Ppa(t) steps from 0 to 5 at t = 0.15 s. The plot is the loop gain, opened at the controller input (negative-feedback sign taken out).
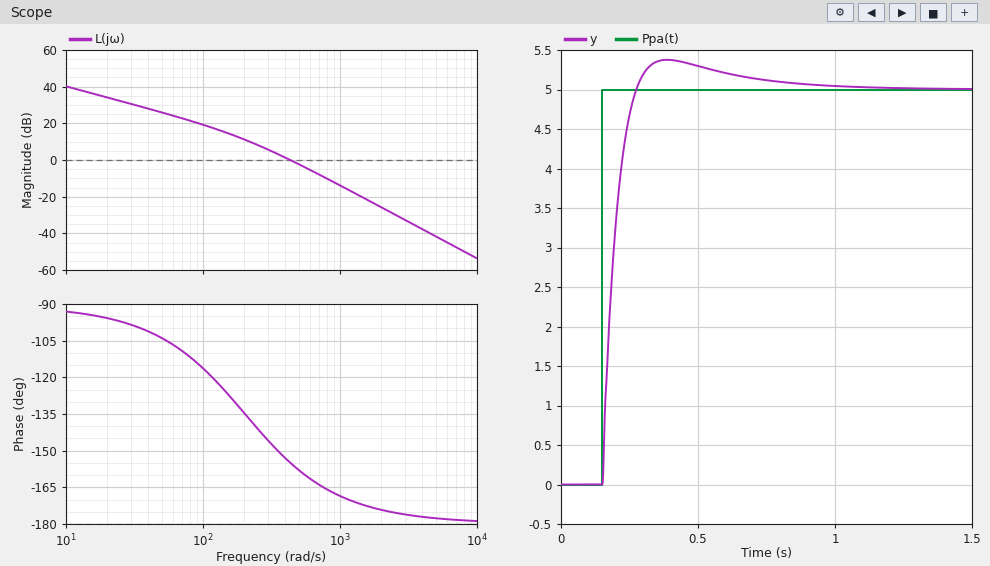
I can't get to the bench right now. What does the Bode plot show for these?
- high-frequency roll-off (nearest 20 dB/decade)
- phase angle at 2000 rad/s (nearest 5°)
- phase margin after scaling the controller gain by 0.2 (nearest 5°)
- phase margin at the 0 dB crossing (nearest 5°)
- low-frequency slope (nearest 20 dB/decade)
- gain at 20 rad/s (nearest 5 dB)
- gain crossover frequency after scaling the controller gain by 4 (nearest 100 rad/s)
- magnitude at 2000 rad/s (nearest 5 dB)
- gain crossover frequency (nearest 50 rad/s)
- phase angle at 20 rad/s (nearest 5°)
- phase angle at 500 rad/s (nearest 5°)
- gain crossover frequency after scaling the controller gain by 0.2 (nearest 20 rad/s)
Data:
-40 dB/decade
-175°
50°
25°
-20 dB/decade
35 dB
900 rad/s
-25 dB
450 rad/s
-95°
-160°
160 rad/s
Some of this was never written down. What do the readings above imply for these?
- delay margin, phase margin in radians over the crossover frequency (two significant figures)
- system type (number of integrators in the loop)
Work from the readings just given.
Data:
0.00097 s
1
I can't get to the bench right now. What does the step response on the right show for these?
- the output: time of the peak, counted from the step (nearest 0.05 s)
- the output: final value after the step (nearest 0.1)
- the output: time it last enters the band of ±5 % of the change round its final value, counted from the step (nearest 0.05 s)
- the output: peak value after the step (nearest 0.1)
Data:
0.25 s
5.0
0.40 s
5.4
